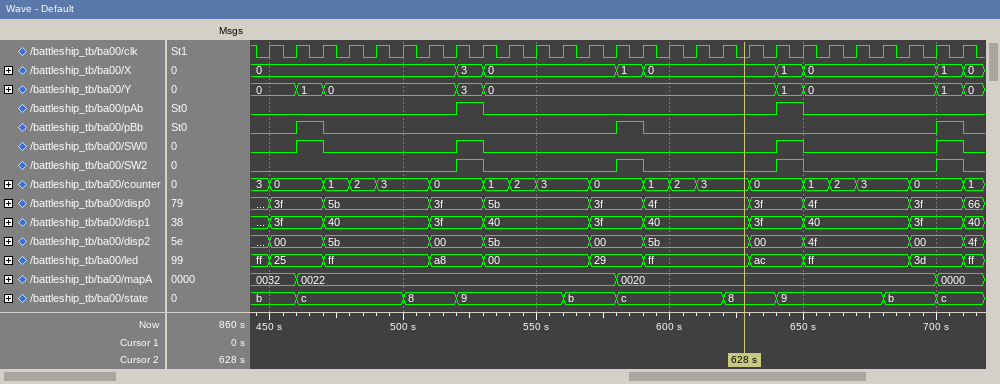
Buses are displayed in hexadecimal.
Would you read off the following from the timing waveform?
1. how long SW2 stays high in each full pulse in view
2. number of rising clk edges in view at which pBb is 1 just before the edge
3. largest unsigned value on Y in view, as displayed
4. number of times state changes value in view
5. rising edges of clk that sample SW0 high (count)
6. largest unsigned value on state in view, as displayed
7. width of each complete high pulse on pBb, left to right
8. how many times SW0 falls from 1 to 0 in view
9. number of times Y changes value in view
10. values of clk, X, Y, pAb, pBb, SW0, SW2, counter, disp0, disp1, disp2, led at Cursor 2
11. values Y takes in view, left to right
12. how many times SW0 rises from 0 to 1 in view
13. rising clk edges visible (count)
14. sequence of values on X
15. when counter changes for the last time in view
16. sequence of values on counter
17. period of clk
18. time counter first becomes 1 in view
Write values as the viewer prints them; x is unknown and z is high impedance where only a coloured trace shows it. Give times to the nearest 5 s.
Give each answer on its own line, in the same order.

10 s, 10 s, 10 s, 10 s
3
3
9
4
c
10 s, 10 s, 10 s
4
8
clk=0, X=0, Y=0, pAb=0, pBb=0, SW0=0, SW2=0, counter=3, disp0=4f, disp1=40, disp2=5b, led=ff
0, 1, 0, 3, 0, 1, 0, 1, 0
4
27
0, 3, 0, 1, 0, 1, 0, 1, 0
710 s
3, 0, 1, 2, 3, 0, 1, 2, 3, 0, 1, 2, 3, 0, 1, 2, 3, 0, 1
10 s
470 s
